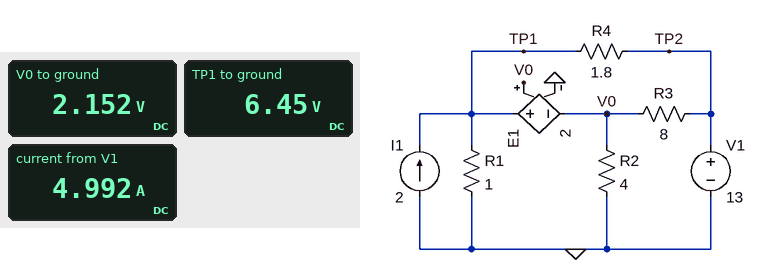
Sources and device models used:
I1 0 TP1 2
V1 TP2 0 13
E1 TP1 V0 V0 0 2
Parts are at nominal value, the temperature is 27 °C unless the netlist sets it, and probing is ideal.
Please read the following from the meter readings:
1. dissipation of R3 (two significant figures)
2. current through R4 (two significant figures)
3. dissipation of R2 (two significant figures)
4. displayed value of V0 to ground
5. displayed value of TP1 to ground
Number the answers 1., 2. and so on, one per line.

1. 15 W
2. 3.6 A
3. 1.2 W
4. 2.152 V
5. 6.45 V
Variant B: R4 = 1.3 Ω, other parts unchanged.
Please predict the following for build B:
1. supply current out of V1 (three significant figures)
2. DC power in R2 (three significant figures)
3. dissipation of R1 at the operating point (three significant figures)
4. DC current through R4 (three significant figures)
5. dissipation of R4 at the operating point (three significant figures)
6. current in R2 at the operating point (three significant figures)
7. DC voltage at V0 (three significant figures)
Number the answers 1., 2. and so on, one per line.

1. 5.79 A
2. 1.44 W
3. 51.7 W
4. 4.47 A
5. 25.9 W
6. 599 mA
7. 2.40 V
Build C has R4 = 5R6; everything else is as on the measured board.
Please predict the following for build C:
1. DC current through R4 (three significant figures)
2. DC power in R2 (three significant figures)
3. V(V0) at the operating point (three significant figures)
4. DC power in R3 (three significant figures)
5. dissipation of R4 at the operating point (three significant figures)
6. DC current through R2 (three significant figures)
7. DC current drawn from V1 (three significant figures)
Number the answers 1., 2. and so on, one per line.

1. 1.51 A
2. 578 mW
3. 1.52 V
4. 16.5 W
5. 12.7 W
6. 380 mA
7. 2.94 A
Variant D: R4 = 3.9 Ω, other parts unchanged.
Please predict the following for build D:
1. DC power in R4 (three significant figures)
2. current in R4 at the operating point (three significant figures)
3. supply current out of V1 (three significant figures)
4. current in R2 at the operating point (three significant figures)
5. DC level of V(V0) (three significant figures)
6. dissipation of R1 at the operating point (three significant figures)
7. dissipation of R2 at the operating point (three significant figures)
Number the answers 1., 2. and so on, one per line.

1. 16.3 W
2. 2.04 A
3. 3.46 A
4. 420 mA
5. 1.68 V
6. 25.4 W
7. 705 mW
